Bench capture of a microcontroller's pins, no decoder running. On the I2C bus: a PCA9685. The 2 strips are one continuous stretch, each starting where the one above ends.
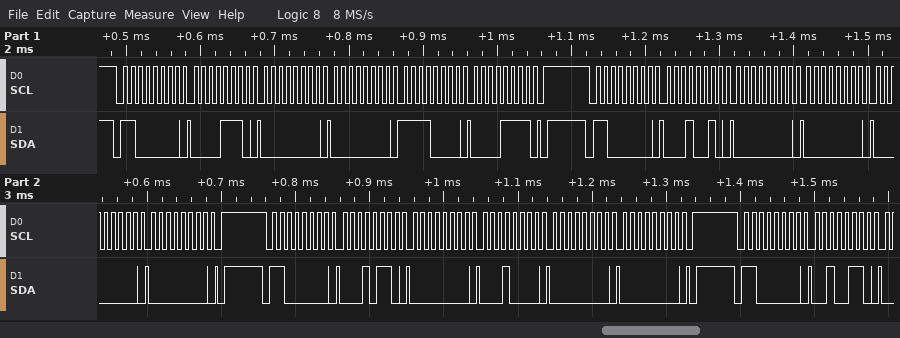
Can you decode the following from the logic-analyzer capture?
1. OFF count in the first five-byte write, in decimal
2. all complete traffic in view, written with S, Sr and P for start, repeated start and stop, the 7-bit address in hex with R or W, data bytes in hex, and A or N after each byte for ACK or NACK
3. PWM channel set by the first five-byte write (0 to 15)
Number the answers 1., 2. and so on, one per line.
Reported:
1. 4080
2. S 60W A 0E A 00 A 00 A F0 A 0F A P S 60W A 12 A 00 A 00 A 00 A 00 A P S 60W A 16 A 00 A 10 A 00 A 00 A P S 60W A 26 A
3. 2
